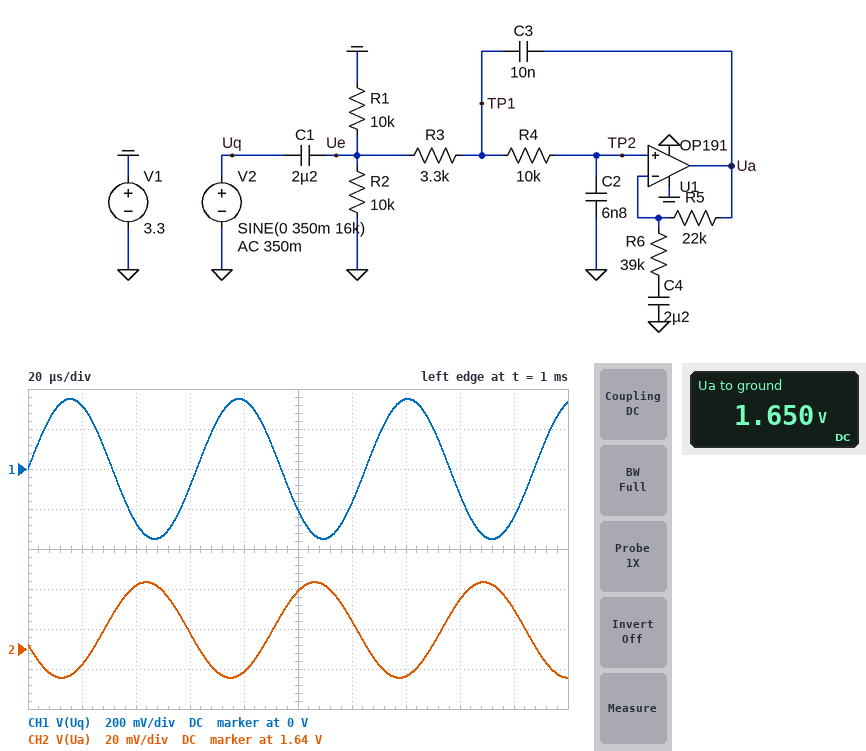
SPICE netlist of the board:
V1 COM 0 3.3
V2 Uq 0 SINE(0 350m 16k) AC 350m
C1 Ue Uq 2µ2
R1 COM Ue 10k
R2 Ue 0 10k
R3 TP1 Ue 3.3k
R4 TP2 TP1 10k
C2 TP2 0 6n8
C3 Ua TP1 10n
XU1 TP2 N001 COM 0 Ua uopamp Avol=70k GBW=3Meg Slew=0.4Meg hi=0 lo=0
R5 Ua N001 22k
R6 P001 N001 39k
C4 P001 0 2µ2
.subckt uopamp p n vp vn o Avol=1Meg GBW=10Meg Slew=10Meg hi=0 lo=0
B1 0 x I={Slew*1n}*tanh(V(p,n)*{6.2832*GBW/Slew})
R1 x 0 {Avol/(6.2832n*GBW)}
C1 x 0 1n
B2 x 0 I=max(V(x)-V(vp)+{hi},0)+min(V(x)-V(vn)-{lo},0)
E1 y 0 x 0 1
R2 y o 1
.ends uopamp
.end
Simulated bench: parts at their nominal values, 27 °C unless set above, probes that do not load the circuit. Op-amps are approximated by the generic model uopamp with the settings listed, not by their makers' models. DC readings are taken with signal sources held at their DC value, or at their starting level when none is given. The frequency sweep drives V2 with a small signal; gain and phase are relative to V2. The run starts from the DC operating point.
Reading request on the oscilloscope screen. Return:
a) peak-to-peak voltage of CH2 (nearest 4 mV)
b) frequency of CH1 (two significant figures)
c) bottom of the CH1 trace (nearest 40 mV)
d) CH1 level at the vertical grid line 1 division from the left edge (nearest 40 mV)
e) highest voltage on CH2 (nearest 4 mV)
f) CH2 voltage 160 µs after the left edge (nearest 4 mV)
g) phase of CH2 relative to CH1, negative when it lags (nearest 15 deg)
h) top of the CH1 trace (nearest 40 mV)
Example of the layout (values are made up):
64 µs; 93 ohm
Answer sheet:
48 mV; 16 kHz; -360 mV; 320 mV; 1.672 V; 1.664 V; -165 deg; 360 mV
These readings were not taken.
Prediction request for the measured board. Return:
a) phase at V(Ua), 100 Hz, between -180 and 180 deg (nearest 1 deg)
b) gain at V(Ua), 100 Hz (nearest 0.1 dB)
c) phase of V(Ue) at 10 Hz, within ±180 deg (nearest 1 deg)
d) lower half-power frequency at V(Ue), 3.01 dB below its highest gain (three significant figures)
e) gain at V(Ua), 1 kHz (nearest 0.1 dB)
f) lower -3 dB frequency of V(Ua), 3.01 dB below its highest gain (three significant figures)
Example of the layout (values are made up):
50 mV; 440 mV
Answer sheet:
6 deg; 3.8 dB; 55 deg; 14.5 Hz; 3.7 dB; 14.5 Hz
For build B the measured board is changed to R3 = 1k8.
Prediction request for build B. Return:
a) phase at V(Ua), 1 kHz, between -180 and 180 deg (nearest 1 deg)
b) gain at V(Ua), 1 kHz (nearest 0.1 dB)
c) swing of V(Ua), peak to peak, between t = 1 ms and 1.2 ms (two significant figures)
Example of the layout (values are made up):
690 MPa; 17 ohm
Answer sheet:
-24 deg; 3.5 dB; 82 mV
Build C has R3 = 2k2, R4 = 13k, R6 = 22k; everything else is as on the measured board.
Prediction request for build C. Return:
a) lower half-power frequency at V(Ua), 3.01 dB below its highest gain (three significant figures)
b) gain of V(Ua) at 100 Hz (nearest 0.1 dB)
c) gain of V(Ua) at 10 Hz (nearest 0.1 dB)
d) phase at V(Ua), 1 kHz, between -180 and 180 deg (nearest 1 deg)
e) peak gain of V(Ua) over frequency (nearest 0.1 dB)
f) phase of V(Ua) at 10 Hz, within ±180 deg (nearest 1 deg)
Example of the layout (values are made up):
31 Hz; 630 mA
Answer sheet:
14.9 Hz; 5.9 dB; 0.8 dB; -28 deg; 6.0 dB; 64 deg
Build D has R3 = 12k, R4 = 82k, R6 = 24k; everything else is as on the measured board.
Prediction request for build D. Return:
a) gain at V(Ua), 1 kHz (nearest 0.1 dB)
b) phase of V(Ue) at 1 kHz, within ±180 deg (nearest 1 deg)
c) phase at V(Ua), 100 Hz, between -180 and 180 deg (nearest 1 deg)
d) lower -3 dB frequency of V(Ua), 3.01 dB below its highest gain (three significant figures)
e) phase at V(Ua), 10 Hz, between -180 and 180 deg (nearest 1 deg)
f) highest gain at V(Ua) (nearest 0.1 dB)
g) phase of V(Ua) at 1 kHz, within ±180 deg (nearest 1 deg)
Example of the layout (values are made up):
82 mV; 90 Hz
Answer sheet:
-5.8 dB; 1 deg; -10 deg; 14.0 Hz; 61 deg; 5.3 dB; -115 deg
